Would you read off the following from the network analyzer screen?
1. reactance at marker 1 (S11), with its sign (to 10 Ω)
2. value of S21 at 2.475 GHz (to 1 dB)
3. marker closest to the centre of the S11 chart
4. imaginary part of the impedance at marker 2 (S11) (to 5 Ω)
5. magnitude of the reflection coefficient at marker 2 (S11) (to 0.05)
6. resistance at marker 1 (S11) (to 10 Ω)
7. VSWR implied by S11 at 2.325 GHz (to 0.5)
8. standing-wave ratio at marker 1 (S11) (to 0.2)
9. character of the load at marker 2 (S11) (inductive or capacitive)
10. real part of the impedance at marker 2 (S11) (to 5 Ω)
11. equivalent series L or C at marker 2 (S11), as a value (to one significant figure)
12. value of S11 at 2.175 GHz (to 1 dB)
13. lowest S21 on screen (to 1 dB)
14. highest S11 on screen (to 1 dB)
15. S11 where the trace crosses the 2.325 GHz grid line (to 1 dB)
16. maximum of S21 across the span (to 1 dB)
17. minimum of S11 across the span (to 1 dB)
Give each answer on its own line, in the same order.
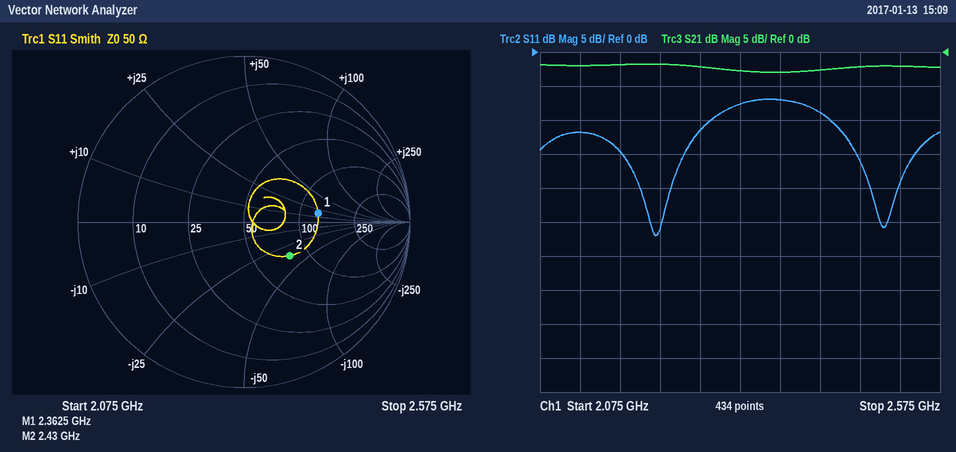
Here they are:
+20 Ω
-2 dB
marker 2
-35 Ω
0.35
130 Ω
2.5
2.6
capacitive
80 Ω
2 pF
-15 dB
-3 dB
-7 dB
-8 dB
-2 dB
-27 dB
